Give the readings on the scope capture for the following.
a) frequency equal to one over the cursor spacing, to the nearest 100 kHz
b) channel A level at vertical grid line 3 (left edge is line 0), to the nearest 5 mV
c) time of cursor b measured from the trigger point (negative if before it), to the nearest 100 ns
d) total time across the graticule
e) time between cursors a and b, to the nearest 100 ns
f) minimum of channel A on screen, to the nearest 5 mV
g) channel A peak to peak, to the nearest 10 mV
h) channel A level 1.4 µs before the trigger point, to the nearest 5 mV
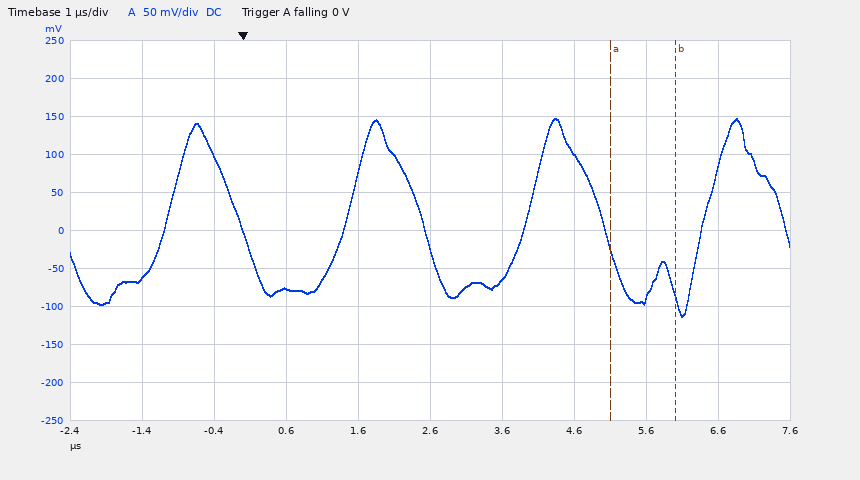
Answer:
1.1 MHz
-75 mV
+6.0 µs
10 µs
900 ns
-115 mV
260 mV
-60 mV
